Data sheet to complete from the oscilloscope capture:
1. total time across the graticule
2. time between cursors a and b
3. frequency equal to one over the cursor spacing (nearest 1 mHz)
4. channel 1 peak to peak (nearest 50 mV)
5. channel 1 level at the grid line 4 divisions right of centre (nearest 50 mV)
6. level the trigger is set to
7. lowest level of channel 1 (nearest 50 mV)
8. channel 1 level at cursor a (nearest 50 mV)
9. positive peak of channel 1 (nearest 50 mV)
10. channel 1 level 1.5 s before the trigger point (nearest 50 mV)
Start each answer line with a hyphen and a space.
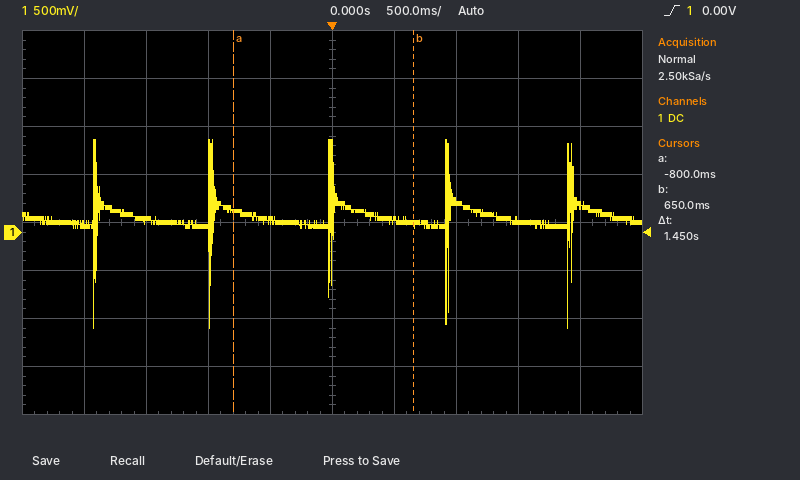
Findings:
- 5 s
- 1.45 s
- 690 mHz
- 1.95 V
- 300 mV
- 0.00 V
- -1.00 V
- 250 mV
- 950 mV
- 100 mV
